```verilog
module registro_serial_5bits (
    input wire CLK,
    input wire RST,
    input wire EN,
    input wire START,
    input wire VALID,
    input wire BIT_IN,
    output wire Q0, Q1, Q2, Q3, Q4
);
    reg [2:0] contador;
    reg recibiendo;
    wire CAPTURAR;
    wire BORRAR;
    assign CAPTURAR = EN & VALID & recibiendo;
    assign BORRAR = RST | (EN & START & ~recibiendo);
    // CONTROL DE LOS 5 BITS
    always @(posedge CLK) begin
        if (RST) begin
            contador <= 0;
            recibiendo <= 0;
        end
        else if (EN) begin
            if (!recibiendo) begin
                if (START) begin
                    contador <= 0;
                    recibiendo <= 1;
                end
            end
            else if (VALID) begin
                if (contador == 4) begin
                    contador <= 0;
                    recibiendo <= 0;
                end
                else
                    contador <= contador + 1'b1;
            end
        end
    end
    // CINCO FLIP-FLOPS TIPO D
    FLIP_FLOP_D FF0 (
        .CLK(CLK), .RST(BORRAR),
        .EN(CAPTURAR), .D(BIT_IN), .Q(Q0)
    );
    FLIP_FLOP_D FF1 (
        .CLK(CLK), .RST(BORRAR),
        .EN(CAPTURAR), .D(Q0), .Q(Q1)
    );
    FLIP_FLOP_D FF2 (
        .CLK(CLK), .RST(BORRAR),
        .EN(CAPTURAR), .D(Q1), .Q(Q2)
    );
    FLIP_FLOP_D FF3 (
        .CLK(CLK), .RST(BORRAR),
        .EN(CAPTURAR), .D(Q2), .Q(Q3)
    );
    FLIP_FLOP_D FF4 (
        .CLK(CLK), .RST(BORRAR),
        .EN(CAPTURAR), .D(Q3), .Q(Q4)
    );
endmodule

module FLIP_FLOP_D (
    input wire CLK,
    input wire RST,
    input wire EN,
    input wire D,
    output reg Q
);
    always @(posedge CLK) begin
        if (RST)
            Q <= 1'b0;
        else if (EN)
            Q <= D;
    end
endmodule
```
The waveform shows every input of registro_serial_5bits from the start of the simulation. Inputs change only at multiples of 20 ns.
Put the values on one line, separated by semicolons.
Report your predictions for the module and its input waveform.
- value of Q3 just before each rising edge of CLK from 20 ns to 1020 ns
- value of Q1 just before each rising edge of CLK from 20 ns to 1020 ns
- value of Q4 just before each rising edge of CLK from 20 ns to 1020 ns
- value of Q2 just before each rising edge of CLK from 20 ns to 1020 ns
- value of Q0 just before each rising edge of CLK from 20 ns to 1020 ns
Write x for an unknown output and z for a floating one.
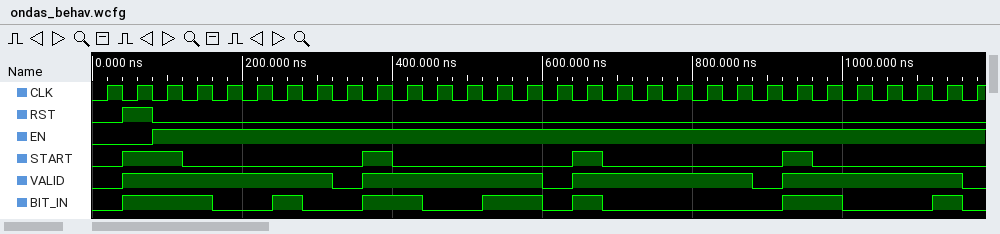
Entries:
x x 0 0 0 0 0 1 0 0 0 0 0 0 1 0 0 0 0 0 0 0 0 0 0 0; x x 0 0 0 1 0 0 1 1 0 0 1 0 0 1 1 0 0 0 0 0 0 0 0 0; x x 0 0 0 0 0 0 1 1 0 0 0 0 0 1 1 0 0 0 0 0 0 0 0 0; x x 0 0 0 0 1 0 0 0 0 0 0 1 0 0 0 0 0 0 0 0 0 0 0 0; x x 0 0 1 0 0 1 0 0 0 1 0 0 1 1 1 0 0 0 0 0 0 0 0 1
